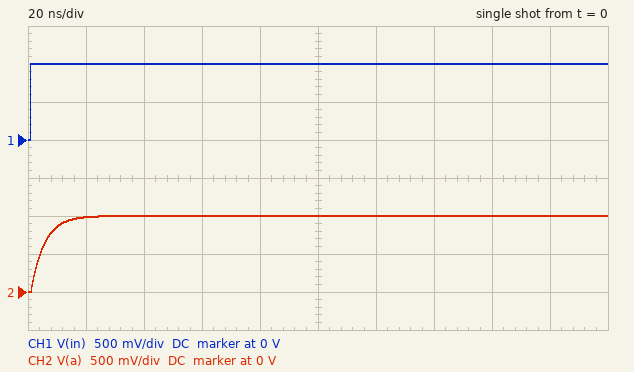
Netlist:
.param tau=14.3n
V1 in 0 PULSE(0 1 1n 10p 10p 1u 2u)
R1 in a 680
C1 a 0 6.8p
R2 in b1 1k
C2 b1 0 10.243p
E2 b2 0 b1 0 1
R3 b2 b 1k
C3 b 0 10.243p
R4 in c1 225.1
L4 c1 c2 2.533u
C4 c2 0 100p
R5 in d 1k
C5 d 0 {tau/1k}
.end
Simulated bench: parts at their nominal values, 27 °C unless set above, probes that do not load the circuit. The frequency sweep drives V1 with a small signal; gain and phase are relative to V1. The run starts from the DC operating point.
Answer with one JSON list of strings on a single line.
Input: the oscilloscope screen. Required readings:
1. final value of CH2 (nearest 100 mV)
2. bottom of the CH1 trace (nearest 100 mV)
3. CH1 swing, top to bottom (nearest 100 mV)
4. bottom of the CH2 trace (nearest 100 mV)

["1.0 V", "0 V", "1.0 V", "0 V"]
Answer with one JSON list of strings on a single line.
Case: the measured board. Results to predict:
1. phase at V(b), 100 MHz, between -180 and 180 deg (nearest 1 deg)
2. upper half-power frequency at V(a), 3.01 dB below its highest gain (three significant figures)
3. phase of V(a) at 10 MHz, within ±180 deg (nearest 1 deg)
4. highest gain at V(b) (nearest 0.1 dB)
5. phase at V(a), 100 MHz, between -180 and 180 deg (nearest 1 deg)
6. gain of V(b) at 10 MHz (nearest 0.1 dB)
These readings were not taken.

["-162 deg", "34.4 MHz", "-16 deg", "0 dB", "-71 deg", "-3.0 dB"]
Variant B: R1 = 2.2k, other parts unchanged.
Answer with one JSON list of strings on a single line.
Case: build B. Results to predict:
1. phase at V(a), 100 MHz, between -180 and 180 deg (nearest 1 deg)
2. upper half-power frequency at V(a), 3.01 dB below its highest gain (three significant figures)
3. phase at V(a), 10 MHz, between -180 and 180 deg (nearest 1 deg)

["-84 deg", "10.6 MHz", "-43 deg"]
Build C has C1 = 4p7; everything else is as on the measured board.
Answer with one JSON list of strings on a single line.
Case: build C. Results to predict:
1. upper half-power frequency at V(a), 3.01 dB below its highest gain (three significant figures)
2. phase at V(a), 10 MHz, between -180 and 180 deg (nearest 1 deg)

["49.8 MHz", "-11 deg"]
